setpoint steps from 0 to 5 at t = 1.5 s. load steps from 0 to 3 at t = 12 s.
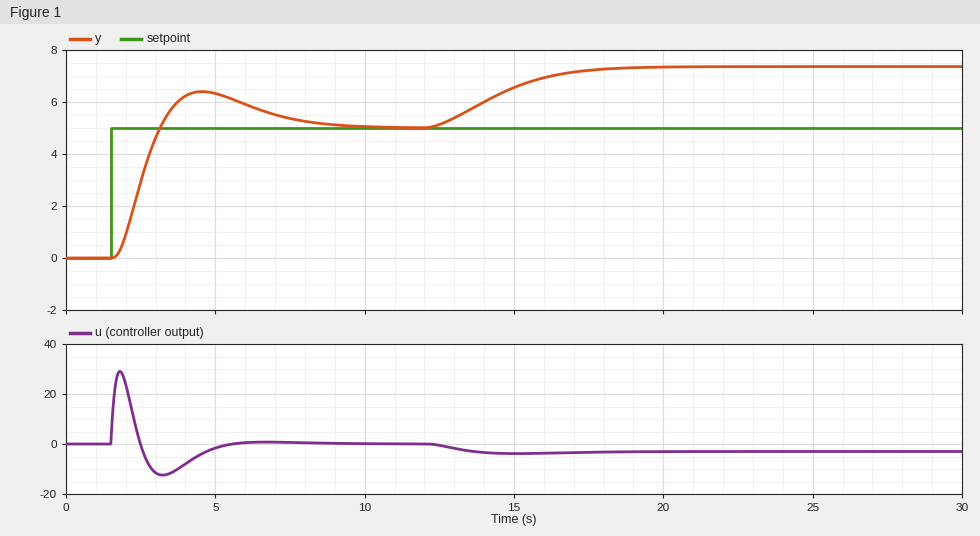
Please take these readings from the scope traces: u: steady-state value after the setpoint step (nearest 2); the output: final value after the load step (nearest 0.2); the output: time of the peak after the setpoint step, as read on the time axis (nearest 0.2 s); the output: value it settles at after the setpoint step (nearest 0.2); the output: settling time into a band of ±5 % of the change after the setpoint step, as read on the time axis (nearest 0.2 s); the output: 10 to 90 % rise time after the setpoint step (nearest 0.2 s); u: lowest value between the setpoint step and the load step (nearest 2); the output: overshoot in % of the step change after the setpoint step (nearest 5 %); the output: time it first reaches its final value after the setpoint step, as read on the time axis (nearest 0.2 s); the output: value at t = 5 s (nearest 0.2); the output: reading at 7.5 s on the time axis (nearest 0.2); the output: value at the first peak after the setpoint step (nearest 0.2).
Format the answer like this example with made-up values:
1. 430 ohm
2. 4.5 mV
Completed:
1. 0
2. 7.4
3. 4.6 s
4. 5.0
5. 8.0 s
6. 1.0 s
7. -12
8. 30 %
9. 3.2 s
10. 6.4
11. 5.4
12. 6.4
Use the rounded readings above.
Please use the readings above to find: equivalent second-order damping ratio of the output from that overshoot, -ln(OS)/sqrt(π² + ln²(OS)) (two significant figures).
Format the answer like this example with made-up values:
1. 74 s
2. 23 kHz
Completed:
1. 0.36
